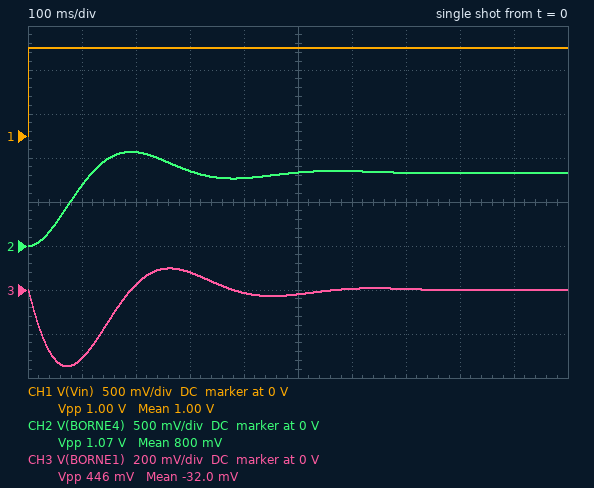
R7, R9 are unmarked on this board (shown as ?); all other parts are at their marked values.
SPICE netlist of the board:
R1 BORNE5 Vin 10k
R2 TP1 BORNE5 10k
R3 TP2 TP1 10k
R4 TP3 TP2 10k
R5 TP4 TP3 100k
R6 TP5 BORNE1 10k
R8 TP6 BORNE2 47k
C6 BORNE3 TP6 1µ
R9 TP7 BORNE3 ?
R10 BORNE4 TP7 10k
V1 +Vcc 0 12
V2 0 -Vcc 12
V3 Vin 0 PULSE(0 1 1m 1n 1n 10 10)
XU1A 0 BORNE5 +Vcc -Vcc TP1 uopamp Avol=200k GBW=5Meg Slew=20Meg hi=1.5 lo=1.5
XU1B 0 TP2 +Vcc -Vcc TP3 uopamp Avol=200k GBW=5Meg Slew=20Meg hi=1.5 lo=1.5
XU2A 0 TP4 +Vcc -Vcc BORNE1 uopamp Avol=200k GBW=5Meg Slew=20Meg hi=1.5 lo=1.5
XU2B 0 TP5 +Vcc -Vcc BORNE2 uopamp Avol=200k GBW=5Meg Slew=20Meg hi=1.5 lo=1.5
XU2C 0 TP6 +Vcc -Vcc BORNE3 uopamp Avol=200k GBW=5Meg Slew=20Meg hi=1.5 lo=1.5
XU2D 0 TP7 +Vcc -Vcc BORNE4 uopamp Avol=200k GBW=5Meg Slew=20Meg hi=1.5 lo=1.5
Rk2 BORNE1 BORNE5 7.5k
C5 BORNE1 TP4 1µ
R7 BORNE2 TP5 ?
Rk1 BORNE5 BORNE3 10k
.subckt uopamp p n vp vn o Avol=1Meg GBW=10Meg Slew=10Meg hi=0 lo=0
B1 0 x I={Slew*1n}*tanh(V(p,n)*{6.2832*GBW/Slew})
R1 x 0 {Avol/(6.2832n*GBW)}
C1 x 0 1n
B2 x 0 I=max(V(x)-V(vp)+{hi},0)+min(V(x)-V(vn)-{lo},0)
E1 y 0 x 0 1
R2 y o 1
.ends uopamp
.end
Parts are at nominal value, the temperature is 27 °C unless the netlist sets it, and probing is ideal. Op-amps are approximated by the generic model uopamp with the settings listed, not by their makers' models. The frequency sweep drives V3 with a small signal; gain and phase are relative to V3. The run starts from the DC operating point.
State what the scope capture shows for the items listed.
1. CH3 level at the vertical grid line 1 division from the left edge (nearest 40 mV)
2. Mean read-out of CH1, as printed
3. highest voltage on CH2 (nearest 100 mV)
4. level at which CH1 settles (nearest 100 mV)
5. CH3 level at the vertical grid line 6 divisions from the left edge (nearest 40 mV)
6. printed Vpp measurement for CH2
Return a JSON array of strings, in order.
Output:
["-320 mV", "1.00 V", "1.1 V", "1.0 V", "0 V", "1.07 V"]
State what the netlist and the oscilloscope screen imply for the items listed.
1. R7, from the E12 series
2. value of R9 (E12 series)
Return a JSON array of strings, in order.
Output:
["15 kΩ", "12 kΩ"]
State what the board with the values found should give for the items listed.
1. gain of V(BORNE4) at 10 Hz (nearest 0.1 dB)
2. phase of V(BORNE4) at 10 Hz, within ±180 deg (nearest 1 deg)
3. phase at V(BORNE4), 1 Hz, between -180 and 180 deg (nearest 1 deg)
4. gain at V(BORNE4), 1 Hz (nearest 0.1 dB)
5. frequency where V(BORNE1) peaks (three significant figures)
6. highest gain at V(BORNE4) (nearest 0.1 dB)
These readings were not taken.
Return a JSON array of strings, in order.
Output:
["-22.9 dB", "-167 deg", "-17 deg", "-0.8 dB", "2.84 Hz", "1.6 dB"]
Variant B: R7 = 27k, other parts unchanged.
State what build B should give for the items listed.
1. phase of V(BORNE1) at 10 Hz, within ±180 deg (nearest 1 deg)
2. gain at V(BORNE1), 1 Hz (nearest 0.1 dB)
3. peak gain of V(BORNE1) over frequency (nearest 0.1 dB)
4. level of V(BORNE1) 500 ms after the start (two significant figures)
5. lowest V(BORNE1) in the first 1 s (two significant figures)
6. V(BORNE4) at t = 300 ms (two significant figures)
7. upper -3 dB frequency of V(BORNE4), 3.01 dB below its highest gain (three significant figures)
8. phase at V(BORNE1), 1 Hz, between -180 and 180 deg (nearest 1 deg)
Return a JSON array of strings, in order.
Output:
["104 deg", "-18.7 dB", "-2.5 dB", "14 mV", "-290 mV", "720 mV", "4.48 Hz", "-99 deg"]
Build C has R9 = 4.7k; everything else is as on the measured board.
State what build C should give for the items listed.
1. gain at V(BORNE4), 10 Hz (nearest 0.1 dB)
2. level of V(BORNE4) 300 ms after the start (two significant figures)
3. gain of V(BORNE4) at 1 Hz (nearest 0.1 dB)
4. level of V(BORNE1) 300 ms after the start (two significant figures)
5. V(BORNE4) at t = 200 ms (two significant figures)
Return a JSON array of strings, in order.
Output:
["-14.8 dB", "2.2 V", "7.3 dB", "80 mV", "2.7 V"]
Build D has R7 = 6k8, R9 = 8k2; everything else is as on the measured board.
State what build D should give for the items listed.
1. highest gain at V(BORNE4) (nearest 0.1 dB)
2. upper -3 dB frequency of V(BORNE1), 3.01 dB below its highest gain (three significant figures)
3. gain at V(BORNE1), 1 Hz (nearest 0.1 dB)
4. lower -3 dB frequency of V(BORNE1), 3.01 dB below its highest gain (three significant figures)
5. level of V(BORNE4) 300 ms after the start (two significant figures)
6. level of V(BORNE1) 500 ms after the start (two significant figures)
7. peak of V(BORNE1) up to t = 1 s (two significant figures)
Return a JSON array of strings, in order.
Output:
["2.4 dB", "3.25 Hz", "-6.6 dB", "1.13 Hz", "1.4 V", "34 mV", "53 mV"]
